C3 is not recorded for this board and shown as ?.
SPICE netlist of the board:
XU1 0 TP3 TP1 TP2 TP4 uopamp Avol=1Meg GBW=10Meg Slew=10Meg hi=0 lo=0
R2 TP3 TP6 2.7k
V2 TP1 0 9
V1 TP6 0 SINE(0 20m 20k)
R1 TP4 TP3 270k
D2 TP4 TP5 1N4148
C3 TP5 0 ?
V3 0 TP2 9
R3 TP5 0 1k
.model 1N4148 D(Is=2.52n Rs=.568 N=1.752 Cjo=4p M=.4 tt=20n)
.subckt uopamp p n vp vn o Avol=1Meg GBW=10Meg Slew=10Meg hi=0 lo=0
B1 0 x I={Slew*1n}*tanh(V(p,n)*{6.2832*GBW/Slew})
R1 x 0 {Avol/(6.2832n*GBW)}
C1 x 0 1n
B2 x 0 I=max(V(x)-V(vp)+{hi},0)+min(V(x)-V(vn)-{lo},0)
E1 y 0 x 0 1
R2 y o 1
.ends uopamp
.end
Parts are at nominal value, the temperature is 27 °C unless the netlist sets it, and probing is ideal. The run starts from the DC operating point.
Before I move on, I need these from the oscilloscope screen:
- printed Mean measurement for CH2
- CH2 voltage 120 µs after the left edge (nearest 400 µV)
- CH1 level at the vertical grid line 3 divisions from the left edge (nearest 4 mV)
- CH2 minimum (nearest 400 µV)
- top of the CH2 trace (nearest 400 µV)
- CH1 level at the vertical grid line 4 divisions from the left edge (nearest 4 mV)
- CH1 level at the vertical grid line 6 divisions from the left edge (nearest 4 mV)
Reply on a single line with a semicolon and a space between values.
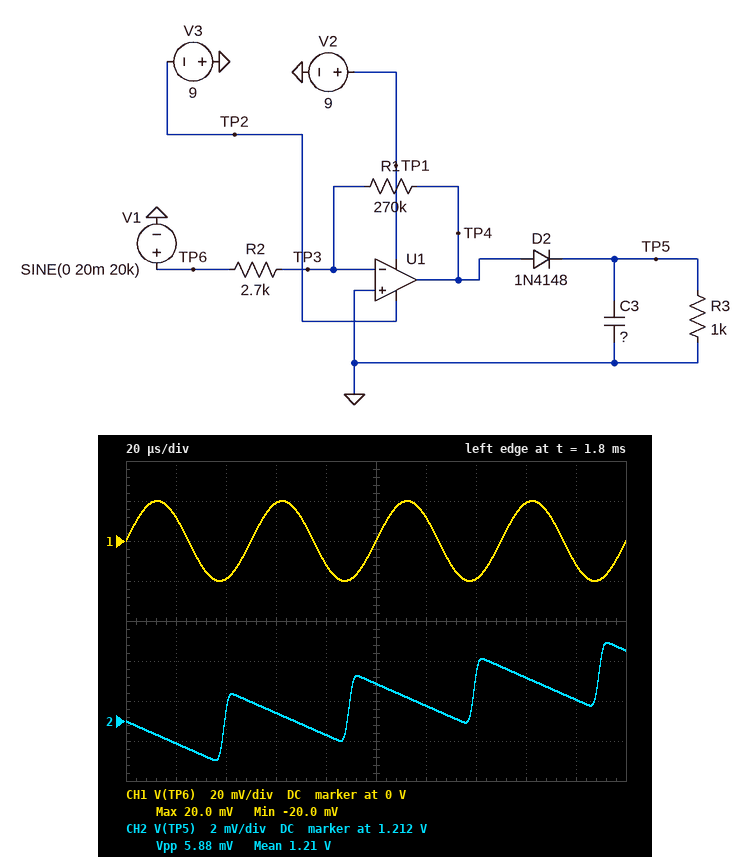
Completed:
1.21 V; 1.2128 V; 20 mV; 1.2100 V; 1.2160 V; -12 mV; 12 mV
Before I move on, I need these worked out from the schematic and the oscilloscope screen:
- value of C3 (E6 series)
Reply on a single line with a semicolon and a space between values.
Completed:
22 µF
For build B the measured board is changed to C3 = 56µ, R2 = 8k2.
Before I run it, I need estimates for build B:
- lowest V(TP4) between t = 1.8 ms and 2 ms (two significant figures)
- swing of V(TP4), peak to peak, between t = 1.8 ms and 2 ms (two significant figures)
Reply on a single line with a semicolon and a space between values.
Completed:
-660 mV; 1.3 V
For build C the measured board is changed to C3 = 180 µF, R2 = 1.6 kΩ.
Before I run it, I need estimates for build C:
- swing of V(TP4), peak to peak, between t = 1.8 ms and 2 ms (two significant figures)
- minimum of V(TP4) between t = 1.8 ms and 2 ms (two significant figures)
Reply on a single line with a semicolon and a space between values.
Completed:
6.3 V; -3.2 V
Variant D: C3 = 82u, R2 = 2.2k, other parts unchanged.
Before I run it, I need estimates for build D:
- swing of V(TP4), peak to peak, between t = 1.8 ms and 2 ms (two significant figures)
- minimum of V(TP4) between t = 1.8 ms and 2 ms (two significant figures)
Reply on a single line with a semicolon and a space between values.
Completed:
4.7 V; -2.4 V
